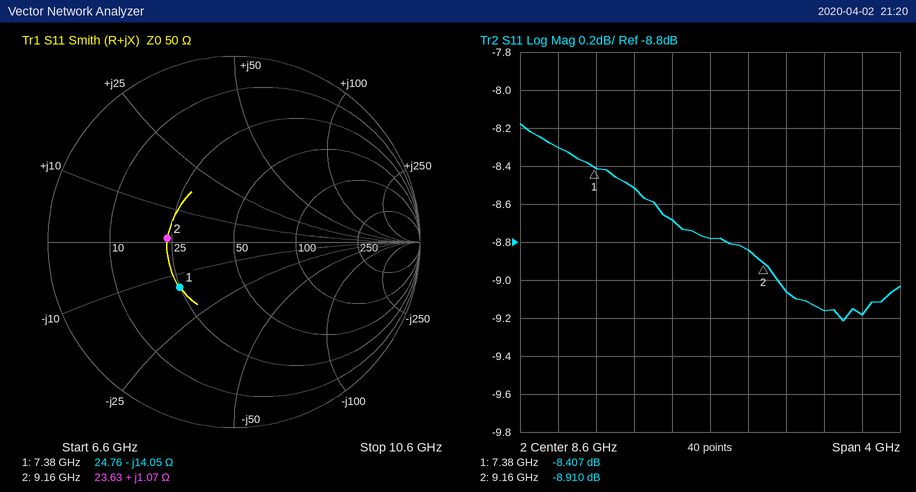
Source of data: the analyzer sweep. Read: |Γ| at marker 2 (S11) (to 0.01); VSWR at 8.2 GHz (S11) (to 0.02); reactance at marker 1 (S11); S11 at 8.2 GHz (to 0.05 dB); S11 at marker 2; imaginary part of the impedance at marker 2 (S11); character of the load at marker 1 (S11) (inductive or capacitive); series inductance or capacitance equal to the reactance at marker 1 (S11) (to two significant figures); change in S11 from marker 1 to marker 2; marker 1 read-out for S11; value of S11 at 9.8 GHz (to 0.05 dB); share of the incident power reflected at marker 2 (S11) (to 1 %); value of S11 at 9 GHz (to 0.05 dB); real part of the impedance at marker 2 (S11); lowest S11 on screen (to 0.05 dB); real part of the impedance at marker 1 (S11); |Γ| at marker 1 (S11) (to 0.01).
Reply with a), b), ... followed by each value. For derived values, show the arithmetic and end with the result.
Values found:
a) 0.36
b) |Γ| = 10^(-8.7/20) = 0.3673; VSWR = (1 + 0.3673)/(1 − 0.3673) ≈ 2.16
c) -14.05 Ω
d) -8.70 dB
e) -8.910 dB
f) +1.07 Ω
g) capacitive
h) C = 1/(2π × 7.38 GHz × 14.05 Ω) ≈ 1.5 pF
i) -8.91 − (-8.407) = -0.503 dB
j) -8.407 dB
k) -9.15 dB
l) 10^(-8.91/10) ≈ 13 %
m) -8.85 dB
n) 23.63 Ω
o) -9.20 dB
p) 24.76 Ω
q) 0.38
